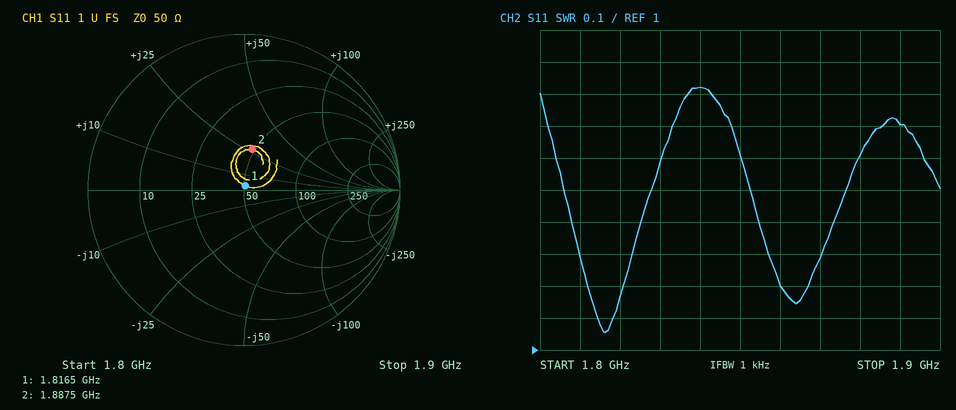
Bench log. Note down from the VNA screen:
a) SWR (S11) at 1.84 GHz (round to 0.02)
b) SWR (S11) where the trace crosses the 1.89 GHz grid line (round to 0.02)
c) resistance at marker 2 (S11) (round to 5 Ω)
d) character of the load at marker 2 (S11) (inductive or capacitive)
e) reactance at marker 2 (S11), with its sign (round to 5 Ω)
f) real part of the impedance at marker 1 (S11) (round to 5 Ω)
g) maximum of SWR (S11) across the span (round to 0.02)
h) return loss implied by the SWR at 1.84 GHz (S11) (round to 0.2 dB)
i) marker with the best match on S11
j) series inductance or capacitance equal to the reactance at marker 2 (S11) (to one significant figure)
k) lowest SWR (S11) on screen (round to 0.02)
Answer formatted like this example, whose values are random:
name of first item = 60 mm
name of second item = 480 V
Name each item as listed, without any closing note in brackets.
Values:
SWR (S11) at 1.84 GHz = 1.82
SWR (S11) where the trace crosses the 1.89 GHz grid line = 1.70
resistance at marker 2 (S11) = 50 Ω
character of the load at marker 2 (S11) = inductive
reactance at marker 2 (S11), with its sign = +25 Ω
real part of the impedance at marker 1 (S11) = 50 Ω
maximum of SWR (S11) across the span = 1.82
return loss implied by the SWR at 1.84 GHz (S11) = 10.8 dB
marker with the best match on S11 = marker 1
series inductance or capacitance equal to the reactance at marker 2 (S11) = 2 nH
lowest SWR (S11) on screen = 1.06
